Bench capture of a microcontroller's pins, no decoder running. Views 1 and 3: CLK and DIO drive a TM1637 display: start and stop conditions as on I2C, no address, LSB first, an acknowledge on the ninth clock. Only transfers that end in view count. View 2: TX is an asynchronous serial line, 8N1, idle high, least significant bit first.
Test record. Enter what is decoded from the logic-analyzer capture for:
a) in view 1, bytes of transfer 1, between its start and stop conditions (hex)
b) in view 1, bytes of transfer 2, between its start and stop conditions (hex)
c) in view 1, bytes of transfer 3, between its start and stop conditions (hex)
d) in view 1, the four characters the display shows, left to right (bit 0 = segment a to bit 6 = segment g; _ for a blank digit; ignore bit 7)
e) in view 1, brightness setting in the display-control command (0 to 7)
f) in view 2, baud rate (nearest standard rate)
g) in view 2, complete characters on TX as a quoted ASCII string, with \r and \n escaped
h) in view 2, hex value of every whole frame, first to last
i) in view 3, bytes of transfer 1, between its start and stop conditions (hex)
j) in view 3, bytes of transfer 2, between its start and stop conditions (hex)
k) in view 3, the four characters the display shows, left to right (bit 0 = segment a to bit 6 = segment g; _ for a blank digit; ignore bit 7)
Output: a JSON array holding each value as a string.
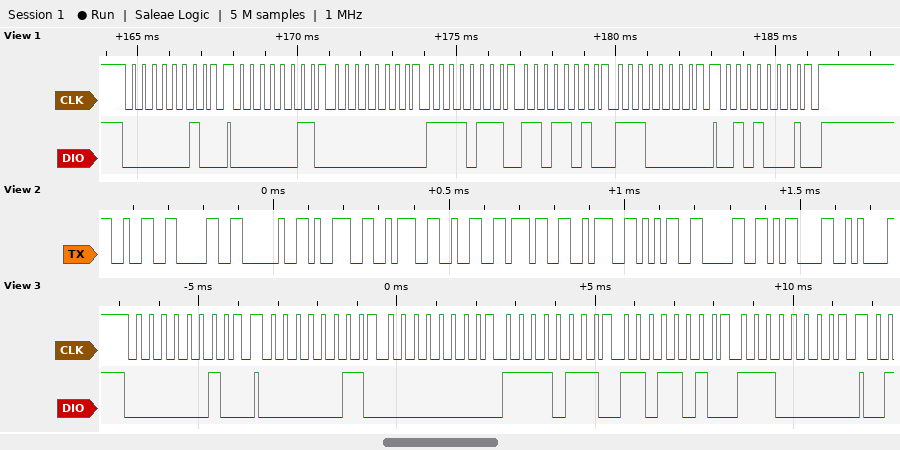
["40", "C0 00 EF 5B 07", "8A", "_927", "2", "57600 baud", "\"20 9:27:50\\r\\n\"", "32 30 20 39 3A 32 37 3A 35 30 0D 0A", "40", "C0 00 EF 5B 07", "_927"]
